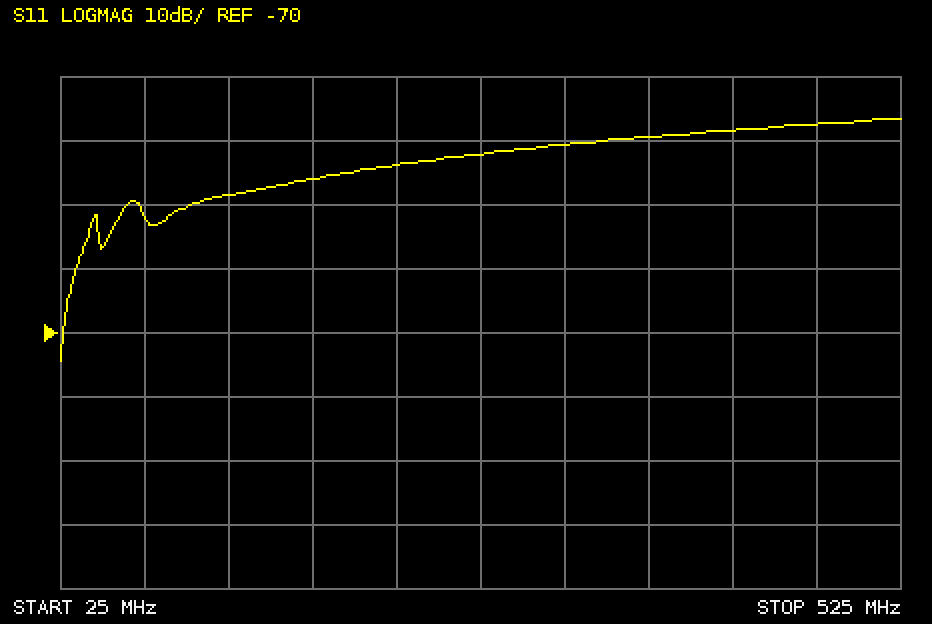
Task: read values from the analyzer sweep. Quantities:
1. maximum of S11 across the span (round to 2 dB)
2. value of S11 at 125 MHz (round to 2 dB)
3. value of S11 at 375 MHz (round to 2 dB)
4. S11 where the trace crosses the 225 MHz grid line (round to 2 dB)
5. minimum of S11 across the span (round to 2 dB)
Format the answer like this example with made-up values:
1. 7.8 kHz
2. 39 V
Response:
1. -36 dB
2. -48 dB
3. -40 dB
4. -44 dB
5. -74 dB
